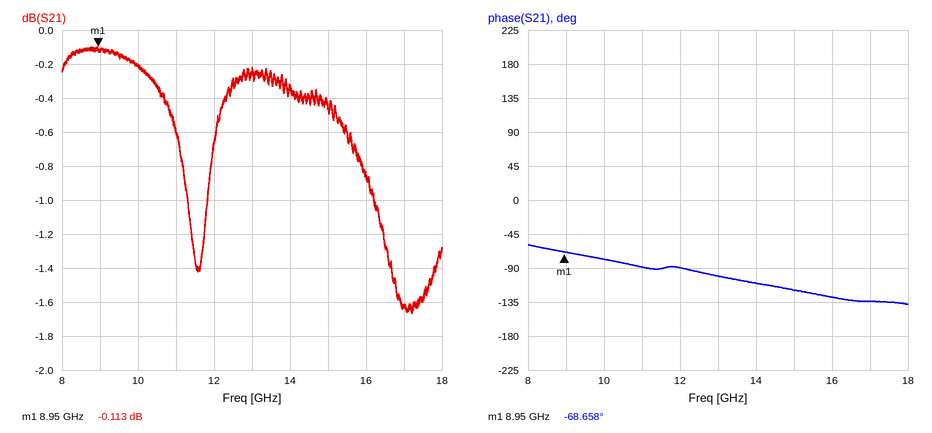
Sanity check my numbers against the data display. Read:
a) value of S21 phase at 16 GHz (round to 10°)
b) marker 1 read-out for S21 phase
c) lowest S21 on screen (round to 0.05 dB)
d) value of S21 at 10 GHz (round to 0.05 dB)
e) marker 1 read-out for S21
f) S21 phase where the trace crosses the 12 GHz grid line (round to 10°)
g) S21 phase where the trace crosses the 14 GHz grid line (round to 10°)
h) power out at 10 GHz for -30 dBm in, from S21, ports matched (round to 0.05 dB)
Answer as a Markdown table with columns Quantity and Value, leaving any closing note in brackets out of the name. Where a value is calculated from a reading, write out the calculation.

| Quantity | Value |
|---|---|
| value of S21 phase at 16 GHz | -130° |
| marker 1 read-out for S21 phase | -68.658° |
| lowest S21 on screen | -1.65 dB |
| value of S21 at 10 GHz | -0.20 dB |
| marker 1 read-out for S21 | -0.113 dB |
| S21 phase where the trace crosses the 12 GHz grid line | -90° |
| S21 phase where the trace crosses the 14 GHz grid line | -110° |
| power out at 10 GHz for -30 dBm in, from S21, ports matched | -30 dBm + (-0.20 dB) = -30.20 dBm |
